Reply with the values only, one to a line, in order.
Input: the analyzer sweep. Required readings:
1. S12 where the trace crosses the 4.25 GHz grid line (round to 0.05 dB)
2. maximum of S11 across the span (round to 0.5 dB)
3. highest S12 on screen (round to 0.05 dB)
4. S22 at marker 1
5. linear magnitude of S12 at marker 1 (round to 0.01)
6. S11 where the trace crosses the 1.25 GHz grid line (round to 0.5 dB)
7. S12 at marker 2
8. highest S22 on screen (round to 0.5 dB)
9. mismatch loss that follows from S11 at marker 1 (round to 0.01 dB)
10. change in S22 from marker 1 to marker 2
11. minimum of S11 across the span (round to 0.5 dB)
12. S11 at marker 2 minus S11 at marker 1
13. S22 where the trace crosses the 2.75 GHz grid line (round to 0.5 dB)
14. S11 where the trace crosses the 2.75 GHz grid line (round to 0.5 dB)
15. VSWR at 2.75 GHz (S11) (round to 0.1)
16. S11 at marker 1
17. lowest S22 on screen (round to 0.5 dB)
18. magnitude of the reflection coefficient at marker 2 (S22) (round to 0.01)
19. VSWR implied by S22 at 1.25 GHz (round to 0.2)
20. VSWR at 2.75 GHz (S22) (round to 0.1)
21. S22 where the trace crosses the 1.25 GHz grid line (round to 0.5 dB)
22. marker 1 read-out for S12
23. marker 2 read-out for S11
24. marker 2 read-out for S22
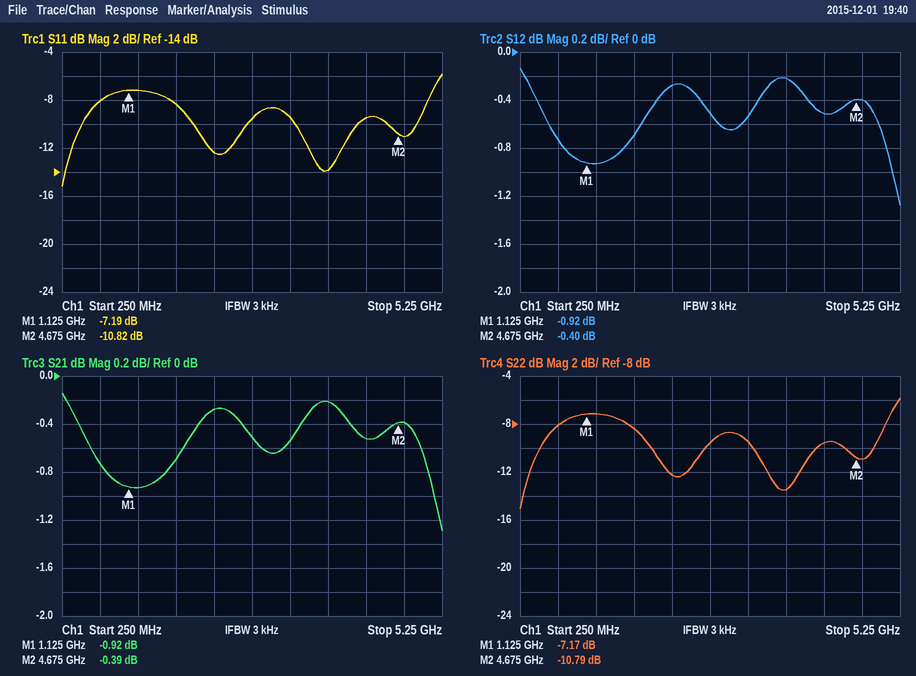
-0.50 dB
-6.0 dB
-0.15 dB
-7.17 dB
0.90
-7.0 dB
-0.40 dB
-6.0 dB
0.92 dB
-3.62 dB
-15.0 dB
-3.63 dB
-9.5 dB
-9.5 dB
2.0
-7.19 dB
-15.0 dB
0.29
2.6
2.0
-7.0 dB
-0.92 dB
-10.82 dB
-10.79 dB
